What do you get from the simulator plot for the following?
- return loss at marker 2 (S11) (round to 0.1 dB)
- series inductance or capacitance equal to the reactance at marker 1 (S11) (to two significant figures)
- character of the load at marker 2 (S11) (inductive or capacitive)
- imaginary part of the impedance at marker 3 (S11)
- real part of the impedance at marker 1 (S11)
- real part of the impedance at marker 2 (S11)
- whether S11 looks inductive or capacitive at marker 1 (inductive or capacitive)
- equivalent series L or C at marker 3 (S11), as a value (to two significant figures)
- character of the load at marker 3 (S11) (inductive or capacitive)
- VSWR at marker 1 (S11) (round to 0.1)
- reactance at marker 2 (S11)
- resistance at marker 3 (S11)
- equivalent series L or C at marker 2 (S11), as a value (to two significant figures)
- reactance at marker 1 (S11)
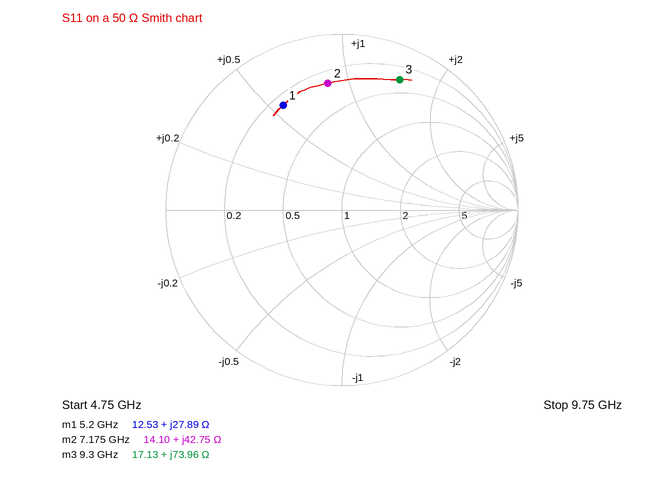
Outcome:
2.8 dB
850 pH
inductive
+73.96 Ω
12.53 Ω
14.10 Ω
inductive
1.3 nH
inductive
5.3
+42.75 Ω
17.13 Ω
950 pH
+27.89 Ω
